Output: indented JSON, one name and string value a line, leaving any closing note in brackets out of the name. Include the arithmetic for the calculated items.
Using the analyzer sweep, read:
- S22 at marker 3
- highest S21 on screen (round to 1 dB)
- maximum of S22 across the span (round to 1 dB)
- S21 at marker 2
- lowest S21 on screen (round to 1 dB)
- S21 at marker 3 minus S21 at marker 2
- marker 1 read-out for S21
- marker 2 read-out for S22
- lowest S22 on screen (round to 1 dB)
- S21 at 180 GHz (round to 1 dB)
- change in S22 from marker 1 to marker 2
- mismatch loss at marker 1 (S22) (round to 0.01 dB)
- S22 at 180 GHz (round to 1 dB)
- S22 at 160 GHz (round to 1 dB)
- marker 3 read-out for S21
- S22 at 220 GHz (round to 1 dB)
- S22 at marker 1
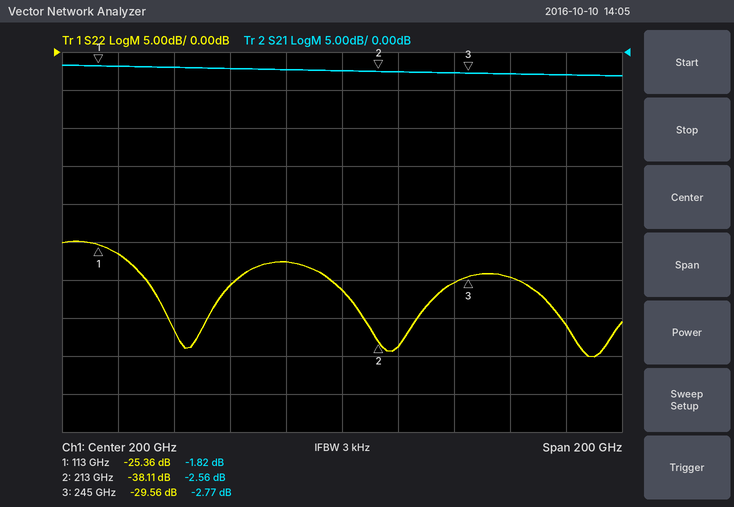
{
  "S22 at marker 3": "-29.56 dB",
  "highest S21 on screen": "-2 dB",
  "maximum of S22 across the span": "-25 dB",
  "S21 at marker 2": "-2.56 dB",
  "lowest S21 on screen": "-3 dB",
  "S21 at marker 3 minus S21 at marker 2": "-2.77 − (-2.56) = -0.21 dB",
  "marker 1 read-out for S21": "-1.82 dB",
  "marker 2 read-out for S22": "-38.11 dB",
  "lowest S22 on screen": "-40 dB",
  "S21 at 180 GHz": "-2 dB",
  "change in S22 from marker 1 to marker 2": "-38.11 − (-25.36) = -12.75 dB",
  "mismatch loss at marker 1 (S22)": "−10 log10(1 − 10^(-25.36/10)) ≈ 0.01 dB",
  "S22 at 180 GHz": "-28 dB",
  "S22 at 160 GHz": "-31 dB",
  "marker 3 read-out for S21": "-2.77 dB",
  "S22 at 220 GHz": "-39 dB",
  "S22 at marker 1": "-25.36 dB"
}
